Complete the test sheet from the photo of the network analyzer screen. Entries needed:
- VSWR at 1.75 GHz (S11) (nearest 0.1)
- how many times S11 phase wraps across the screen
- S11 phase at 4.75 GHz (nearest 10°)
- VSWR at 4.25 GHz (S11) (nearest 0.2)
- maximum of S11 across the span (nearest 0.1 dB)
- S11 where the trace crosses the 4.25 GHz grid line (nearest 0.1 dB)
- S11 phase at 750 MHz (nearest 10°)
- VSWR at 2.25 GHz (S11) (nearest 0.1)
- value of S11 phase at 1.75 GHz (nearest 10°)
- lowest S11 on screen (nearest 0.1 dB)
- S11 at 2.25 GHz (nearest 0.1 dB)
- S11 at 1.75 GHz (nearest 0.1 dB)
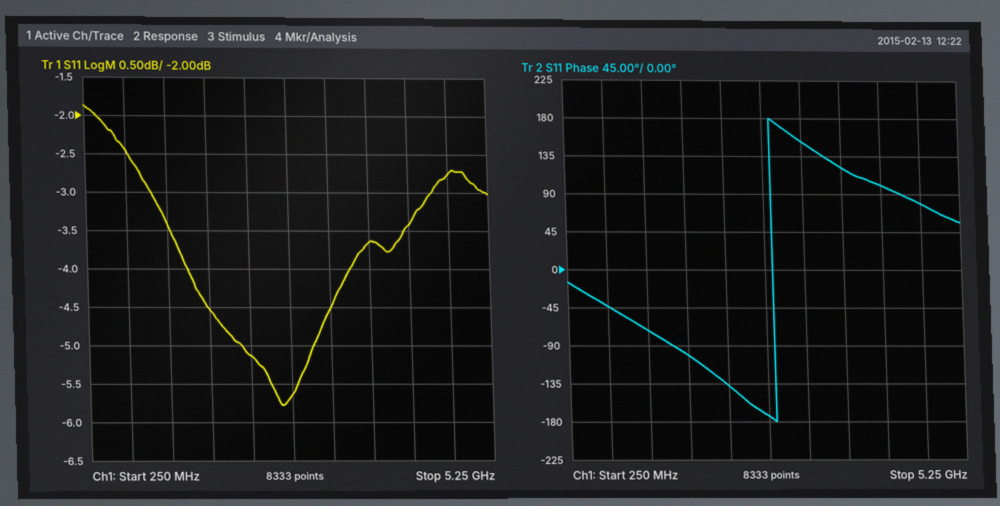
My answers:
3.9
1
80°
5.2
-1.9 dB
-3.4 dB
-40°
3.5
-100°
-5.8 dB
-5.1 dB
-4.5 dB
